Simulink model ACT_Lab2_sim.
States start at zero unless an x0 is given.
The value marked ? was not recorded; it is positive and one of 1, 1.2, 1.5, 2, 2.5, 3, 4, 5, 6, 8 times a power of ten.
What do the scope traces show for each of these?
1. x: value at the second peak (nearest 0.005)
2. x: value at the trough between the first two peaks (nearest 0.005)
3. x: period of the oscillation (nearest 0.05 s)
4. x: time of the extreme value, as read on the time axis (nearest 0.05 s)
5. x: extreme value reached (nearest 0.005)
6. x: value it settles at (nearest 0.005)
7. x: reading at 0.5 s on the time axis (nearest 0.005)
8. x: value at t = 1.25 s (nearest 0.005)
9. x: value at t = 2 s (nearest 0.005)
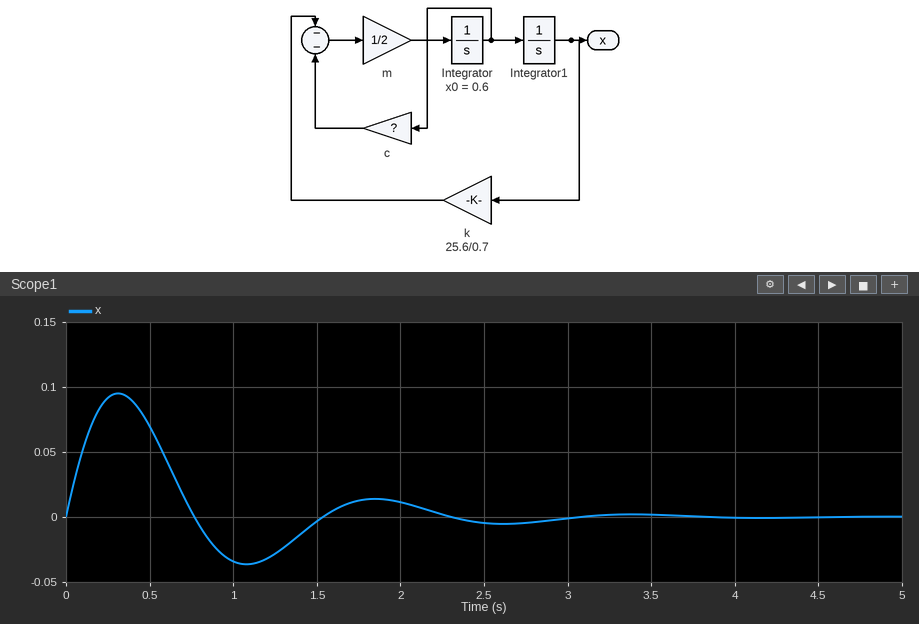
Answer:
0.015
-0.035
1.55 s
0.30 s
0.095
0.000
0.070
-0.030
0.010
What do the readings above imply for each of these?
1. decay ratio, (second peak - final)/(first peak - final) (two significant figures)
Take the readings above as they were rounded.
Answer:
0.16
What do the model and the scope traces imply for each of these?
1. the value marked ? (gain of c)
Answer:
5
